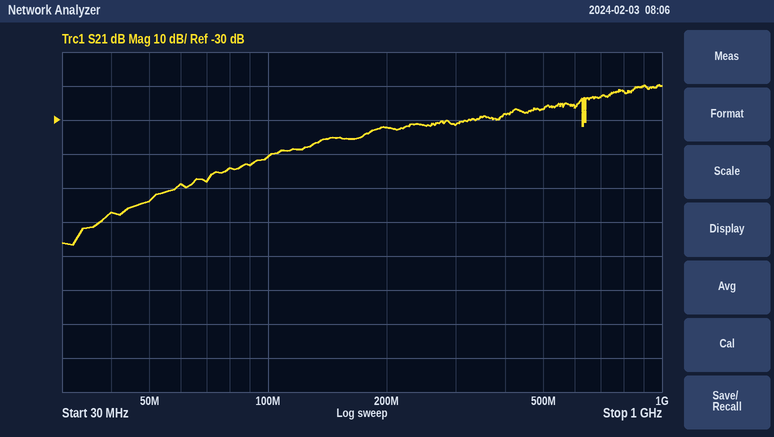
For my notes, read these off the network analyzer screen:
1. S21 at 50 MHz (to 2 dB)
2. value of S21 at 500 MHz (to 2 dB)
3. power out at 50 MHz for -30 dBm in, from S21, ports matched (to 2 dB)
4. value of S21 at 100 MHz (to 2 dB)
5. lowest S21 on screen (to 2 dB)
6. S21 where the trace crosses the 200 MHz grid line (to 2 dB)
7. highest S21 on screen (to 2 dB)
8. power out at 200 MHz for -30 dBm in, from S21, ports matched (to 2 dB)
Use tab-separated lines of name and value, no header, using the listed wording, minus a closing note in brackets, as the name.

S21 at 50 MHz	-54 dB
value of S21 at 500 MHz	-26 dB
power out at 50 MHz for -30 dBm in, from S21, ports matched	-84 dBm
value of S21 at 100 MHz	-40 dB
lowest S21 on screen	-66 dB
S21 where the trace crosses the 200 MHz grid line	-32 dB
highest S21 on screen	-20 dB
power out at 200 MHz for -30 dBm in, from S21, ports matched	-62 dBm
